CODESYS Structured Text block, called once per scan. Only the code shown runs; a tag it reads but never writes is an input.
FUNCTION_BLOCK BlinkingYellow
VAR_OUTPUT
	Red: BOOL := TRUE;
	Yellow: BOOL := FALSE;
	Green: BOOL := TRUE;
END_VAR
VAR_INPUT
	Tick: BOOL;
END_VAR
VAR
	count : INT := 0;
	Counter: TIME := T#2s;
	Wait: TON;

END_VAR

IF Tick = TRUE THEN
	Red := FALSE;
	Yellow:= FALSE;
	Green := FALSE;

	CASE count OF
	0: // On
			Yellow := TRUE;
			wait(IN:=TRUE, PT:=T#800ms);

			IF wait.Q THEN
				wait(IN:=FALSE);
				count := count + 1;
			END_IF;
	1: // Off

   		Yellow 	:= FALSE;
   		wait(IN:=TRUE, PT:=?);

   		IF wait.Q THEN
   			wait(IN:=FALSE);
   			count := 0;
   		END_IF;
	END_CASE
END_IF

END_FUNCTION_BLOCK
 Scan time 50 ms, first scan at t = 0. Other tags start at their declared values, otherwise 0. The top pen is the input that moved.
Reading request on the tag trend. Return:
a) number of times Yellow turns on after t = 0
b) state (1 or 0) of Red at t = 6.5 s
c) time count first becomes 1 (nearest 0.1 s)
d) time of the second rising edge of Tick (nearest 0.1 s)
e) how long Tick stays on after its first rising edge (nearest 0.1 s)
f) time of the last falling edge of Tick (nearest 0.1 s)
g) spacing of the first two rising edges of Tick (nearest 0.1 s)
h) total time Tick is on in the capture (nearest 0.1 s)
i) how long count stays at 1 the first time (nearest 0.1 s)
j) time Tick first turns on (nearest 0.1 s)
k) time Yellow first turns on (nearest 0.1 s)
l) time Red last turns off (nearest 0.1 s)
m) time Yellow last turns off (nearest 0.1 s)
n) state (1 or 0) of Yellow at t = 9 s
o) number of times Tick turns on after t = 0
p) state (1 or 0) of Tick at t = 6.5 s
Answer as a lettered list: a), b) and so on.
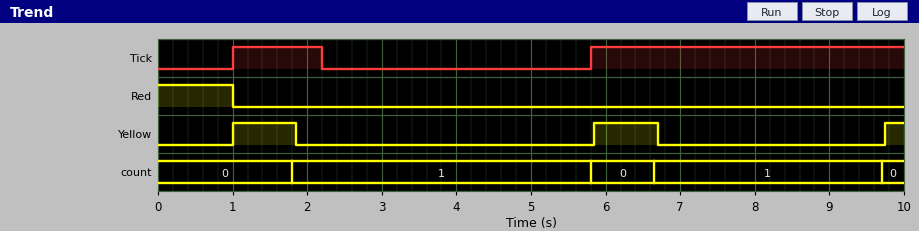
a) 3
b) 0
c) 1.8 s
d) 5.8 s
e) 1.2 s
f) 2.2 s
g) 4.8 s
h) 5.4 s
i) 4.0 s
j) 1.0 s
k) 1.0 s
l) 1.0 s
m) 6.7 s
n) 0
o) 2
p) 1
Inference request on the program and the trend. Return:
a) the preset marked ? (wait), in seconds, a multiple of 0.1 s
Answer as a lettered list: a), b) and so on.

a) 3.0 s
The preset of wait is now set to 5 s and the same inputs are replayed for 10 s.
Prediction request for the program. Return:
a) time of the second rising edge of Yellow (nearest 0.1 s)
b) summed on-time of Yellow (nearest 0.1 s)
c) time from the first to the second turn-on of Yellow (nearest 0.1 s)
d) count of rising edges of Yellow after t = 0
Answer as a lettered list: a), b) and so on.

a) 6.9 s
b) 1.7 s
c) 5.9 s
d) 2
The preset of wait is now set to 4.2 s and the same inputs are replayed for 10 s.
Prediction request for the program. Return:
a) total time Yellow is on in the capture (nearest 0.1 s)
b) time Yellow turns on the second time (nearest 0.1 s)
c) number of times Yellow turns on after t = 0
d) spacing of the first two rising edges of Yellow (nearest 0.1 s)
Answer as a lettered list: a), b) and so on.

a) 1.7 s
b) 6.1 s
c) 2
d) 5.1 s
